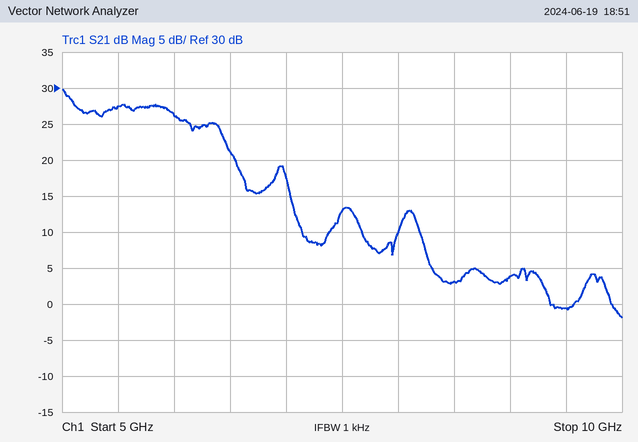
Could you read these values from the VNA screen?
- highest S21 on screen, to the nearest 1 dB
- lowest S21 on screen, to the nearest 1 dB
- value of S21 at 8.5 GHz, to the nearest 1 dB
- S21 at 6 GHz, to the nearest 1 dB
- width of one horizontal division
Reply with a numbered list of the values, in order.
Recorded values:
1. 30 dB
2. -2 dB
3. 3 dB
4. 26 dB
5. 500 MHz
